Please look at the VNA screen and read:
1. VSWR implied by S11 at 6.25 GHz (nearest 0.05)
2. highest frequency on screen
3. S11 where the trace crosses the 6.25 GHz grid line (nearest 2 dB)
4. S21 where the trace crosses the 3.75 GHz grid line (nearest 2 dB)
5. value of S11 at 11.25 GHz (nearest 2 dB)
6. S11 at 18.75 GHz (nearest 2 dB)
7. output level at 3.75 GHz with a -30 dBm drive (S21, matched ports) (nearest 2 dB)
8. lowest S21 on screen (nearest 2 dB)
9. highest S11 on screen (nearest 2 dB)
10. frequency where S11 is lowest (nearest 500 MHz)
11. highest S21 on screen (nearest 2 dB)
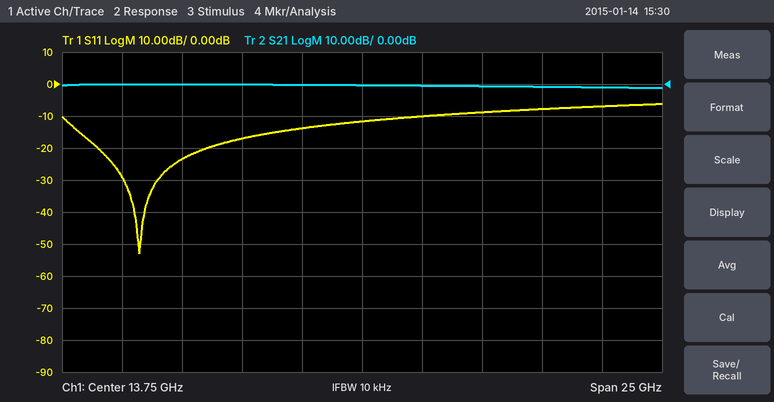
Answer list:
1.15
26.25 GHz
-24 dB
0 dB
-14 dB
-8 dB
-30 dBm
-2 dB
-6 dB
4.5 GHz
0 dB
